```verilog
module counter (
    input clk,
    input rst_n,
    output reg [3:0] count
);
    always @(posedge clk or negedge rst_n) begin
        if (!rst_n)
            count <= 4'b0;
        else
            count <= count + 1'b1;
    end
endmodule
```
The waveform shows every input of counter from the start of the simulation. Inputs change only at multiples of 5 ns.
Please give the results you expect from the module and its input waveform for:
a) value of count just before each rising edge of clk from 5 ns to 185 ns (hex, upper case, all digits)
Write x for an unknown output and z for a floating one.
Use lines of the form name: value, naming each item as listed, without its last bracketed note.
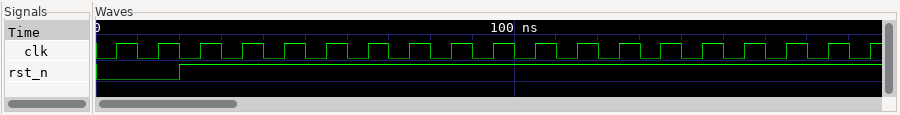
value of count just before each rising edge of clk from 5 ns to 185 ns: 0, 0, 0, 1, 2, 3, 4, 5, 6, 7, 8, 9, A, B, C, D, E, F, 0
